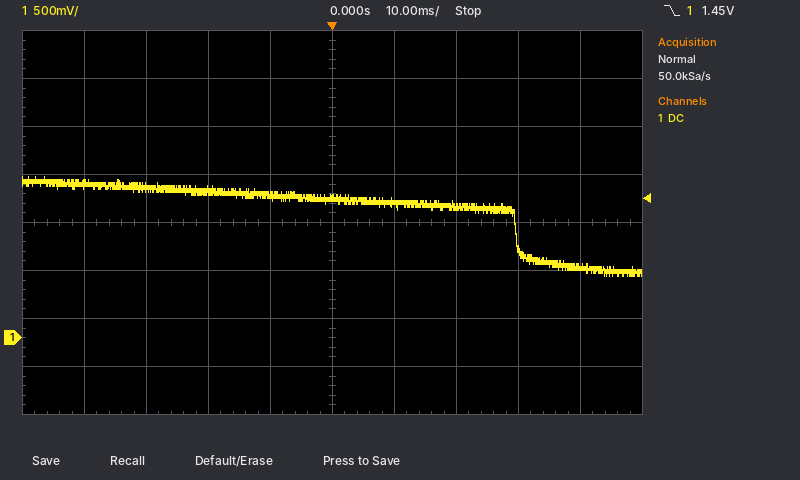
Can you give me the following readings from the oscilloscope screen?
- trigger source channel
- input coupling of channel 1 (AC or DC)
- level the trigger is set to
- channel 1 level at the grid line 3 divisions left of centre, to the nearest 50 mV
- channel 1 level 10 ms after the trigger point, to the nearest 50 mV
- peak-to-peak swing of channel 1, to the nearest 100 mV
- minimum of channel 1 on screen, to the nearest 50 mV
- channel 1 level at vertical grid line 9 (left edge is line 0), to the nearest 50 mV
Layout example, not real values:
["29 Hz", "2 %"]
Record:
["channel 1", "DC", "1.45 V", "1.55 V", "1.40 V", "1.00 V", "650 mV", "750 mV"]
